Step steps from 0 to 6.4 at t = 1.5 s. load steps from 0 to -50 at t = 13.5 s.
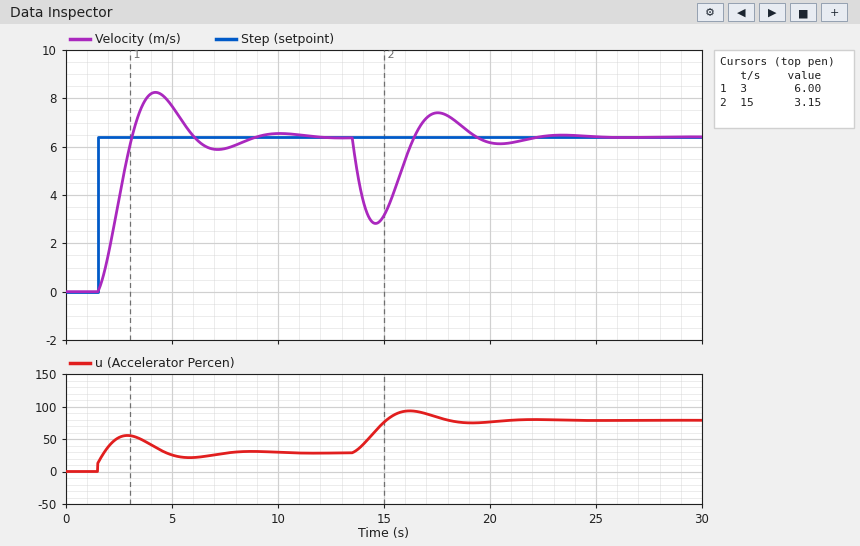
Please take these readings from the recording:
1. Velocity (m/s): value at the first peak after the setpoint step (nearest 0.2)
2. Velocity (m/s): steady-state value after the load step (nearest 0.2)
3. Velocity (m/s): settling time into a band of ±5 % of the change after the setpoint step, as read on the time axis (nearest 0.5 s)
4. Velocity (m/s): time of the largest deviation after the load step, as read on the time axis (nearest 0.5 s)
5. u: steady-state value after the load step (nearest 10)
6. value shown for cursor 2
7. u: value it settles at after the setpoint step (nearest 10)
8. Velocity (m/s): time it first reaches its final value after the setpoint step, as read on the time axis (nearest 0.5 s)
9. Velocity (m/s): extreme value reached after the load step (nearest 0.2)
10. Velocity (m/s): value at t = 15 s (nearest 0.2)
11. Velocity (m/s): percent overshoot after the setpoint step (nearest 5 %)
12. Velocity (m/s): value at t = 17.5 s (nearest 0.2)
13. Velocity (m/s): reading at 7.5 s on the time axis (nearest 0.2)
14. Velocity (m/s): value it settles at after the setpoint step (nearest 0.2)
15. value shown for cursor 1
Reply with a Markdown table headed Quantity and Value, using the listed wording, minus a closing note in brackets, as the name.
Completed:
| Quantity | Value |
|---|---|
| Velocity (m/s): value at the first peak after the setpoint step | 8.2 |
| Velocity (m/s): steady-state value after the load step | 6.4 |
| Velocity (m/s): settling time into a band of ±5 % of the change after the setpoint step, as read on the time axis | 8.0 s |
| Velocity (m/s): time of the largest deviation after the load step, as read on the time axis | 14.5 s |
| u: steady-state value after the load step | 80 |
| value shown for cursor 2 | 3.15 |
| u: value it settles at after the setpoint step | 30 |
| Velocity (m/s): time it first reaches its final value after the setpoint step, as read on the time axis | 3.0 s |
| Velocity (m/s): extreme value reached after the load step | 2.8 |
| Velocity (m/s): value at t = 15 s | 3.2 |
| Velocity (m/s): percent overshoot after the setpoint step | 30 % |
| Velocity (m/s): value at t = 17.5 s | 7.4 |
| Velocity (m/s): reading at 7.5 s on the time axis | 6.0 |
| Velocity (m/s): value it settles at after the setpoint step | 6.4 |
| value shown for cursor 1 | 6.00 |
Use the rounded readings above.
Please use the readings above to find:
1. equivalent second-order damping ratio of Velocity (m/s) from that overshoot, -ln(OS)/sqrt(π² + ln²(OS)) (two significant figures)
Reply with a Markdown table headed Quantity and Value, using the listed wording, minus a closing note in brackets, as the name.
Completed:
| Quantity | Value |
|---|---|
| equivalent second-order damping ratio of Velocity (m/s) from that overshoot, -ln(OS)/sqrt(π² + ln²(OS)) | 0.36 |
